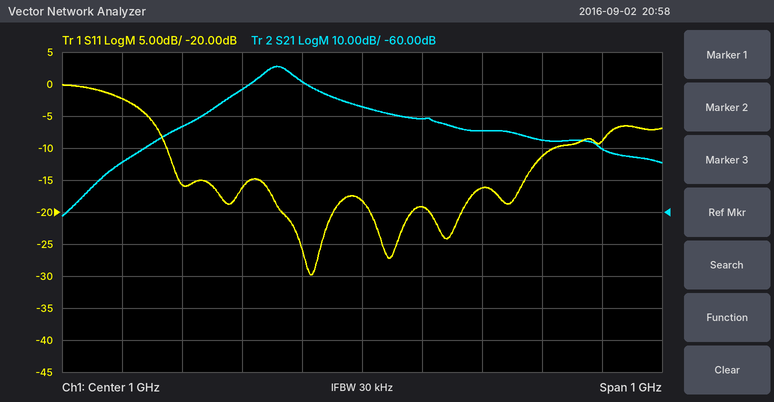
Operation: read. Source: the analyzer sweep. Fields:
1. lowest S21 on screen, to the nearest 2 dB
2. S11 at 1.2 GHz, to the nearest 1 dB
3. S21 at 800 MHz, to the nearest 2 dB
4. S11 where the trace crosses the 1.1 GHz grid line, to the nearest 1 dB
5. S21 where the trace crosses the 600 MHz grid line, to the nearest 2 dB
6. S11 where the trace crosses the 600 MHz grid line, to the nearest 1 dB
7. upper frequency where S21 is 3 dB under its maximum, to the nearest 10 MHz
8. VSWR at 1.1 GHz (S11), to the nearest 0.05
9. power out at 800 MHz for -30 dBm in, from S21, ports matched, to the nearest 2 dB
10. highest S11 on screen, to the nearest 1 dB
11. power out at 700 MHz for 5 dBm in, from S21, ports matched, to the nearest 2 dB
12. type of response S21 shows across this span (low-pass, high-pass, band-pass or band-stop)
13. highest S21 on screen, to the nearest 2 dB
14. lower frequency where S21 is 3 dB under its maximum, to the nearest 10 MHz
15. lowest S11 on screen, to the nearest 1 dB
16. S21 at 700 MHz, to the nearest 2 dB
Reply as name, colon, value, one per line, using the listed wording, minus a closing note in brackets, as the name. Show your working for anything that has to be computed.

lowest S21 on screen, to the nearest 2 dB: -62 dB
S11 at 1.2 GHz, to the nearest 1 dB: -16 dB
S21 at 800 MHz, to the nearest 2 dB: -22 dB
S11 where the trace crosses the 1.1 GHz grid line, to the nearest 1 dB: -19 dB
S21 where the trace crosses the 600 MHz grid line, to the nearest 2 dB: -44 dB
S11 where the trace crosses the 600 MHz grid line, to the nearest 1 dB: -2 dB
upper frequency where S21 is 3 dB under its maximum, to the nearest 10 MHz: 890 MHz
VSWR at 1.1 GHz (S11), to the nearest 0.05: |Γ| = 10^(-19/20) = 0.1122; VSWR = (1 + 0.1122)/(1 − 0.1122) ≈ 1.25
power out at 800 MHz for -30 dBm in, from S21, ports matched, to the nearest 2 dB: -30 dBm + (-22 dB) = -52 dBm
highest S11 on screen, to the nearest 1 dB: 0 dB
power out at 700 MHz for 5 dBm in, from S21, ports matched, to the nearest 2 dB: 5 dBm + (-34 dB) = -28 dBm
type of response S21 shows across this span: band-pass
highest S21 on screen, to the nearest 2 dB: -14 dB
lower frequency where S21 is 3 dB under its maximum, to the nearest 10 MHz: 830 MHz
lowest S11 on screen, to the nearest 1 dB: -30 dB
S21 at 700 MHz, to the nearest 2 dB: -34 dB
